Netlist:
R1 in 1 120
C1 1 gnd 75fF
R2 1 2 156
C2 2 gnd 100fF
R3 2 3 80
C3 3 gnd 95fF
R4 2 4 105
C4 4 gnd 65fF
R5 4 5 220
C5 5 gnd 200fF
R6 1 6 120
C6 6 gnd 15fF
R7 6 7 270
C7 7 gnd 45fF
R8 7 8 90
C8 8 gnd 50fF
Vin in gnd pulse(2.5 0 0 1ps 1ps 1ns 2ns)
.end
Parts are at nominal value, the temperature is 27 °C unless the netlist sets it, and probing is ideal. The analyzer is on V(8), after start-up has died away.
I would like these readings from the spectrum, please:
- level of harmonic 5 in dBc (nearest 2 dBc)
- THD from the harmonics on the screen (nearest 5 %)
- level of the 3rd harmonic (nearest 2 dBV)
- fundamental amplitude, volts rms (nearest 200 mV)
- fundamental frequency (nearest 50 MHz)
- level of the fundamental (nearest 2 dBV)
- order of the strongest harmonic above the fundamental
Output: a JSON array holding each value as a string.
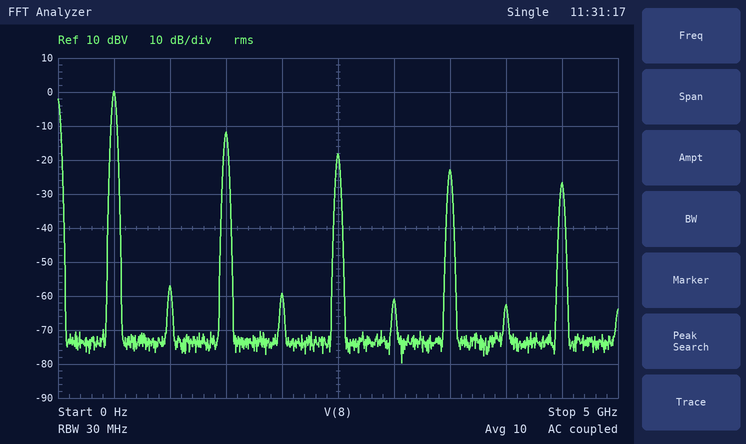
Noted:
["-18 dBc", "30 %", "-12 dBV", "1.0 V", "500 MHz", "0 dBV", "3"]
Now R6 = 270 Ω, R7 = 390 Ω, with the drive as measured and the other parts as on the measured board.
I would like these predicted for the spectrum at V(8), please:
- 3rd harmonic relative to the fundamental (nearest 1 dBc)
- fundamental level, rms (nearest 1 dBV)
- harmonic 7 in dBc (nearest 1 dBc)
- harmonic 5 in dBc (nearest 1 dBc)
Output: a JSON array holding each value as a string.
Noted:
["-13 dBc", "0 dBV", "-25 dBc", "-20 dBc"]
